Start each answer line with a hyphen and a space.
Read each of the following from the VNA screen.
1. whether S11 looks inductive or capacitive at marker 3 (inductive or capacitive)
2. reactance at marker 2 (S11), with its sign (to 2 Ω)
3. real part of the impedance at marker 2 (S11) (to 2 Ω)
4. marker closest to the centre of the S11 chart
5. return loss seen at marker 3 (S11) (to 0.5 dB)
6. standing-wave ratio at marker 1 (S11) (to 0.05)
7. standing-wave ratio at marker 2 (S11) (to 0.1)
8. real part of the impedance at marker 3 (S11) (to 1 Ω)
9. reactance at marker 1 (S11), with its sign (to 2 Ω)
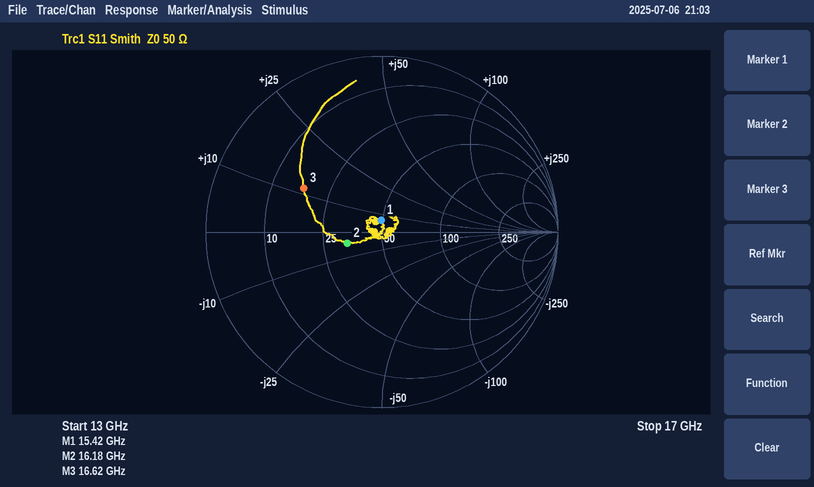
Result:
- inductive
- -4 Ω
- 34 Ω
- marker 1
- 6.0 dB
- 1.15
- 1.5
- 17 Ω
- +6 Ω
